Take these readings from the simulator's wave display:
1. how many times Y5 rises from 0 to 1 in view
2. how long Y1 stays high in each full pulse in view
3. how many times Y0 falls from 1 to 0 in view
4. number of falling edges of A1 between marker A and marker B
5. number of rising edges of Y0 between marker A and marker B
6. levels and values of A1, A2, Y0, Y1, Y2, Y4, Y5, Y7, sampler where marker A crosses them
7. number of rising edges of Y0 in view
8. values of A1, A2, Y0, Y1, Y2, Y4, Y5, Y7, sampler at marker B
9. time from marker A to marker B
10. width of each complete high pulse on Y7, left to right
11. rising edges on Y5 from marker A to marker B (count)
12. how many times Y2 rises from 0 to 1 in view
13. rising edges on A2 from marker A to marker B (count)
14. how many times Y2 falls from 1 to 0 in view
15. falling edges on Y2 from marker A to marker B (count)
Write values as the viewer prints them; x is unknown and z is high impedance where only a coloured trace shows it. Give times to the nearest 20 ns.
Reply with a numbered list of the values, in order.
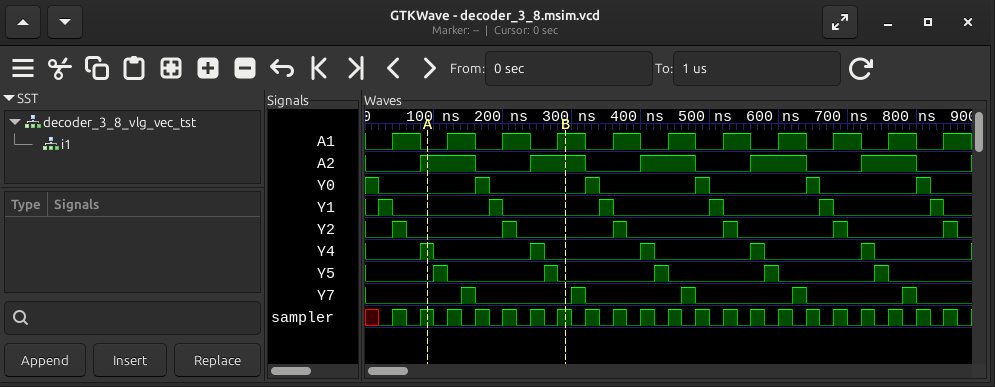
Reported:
1. 5
2. 20 ns, 20 ns, 20 ns, 20 ns, 20 ns, 20 ns
3. 6
4. 2
5. 1
6. A1=0, A2=1, Y0=0, Y1=0, Y2=0, Y4=1, Y5=0, Y7=0, sampler=1
7. 5
8. A1=1, A2=1, Y0=0, Y1=0, Y2=0, Y4=0, Y5=0, Y7=0, sampler=1
9. 200 ns
10. 20 ns, 20 ns, 20 ns, 20 ns, 20 ns
11. 2
12. 6
13. 1
14. 6
15. 1
